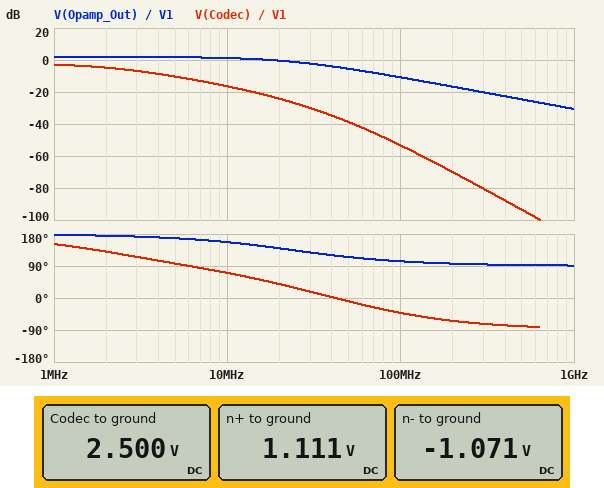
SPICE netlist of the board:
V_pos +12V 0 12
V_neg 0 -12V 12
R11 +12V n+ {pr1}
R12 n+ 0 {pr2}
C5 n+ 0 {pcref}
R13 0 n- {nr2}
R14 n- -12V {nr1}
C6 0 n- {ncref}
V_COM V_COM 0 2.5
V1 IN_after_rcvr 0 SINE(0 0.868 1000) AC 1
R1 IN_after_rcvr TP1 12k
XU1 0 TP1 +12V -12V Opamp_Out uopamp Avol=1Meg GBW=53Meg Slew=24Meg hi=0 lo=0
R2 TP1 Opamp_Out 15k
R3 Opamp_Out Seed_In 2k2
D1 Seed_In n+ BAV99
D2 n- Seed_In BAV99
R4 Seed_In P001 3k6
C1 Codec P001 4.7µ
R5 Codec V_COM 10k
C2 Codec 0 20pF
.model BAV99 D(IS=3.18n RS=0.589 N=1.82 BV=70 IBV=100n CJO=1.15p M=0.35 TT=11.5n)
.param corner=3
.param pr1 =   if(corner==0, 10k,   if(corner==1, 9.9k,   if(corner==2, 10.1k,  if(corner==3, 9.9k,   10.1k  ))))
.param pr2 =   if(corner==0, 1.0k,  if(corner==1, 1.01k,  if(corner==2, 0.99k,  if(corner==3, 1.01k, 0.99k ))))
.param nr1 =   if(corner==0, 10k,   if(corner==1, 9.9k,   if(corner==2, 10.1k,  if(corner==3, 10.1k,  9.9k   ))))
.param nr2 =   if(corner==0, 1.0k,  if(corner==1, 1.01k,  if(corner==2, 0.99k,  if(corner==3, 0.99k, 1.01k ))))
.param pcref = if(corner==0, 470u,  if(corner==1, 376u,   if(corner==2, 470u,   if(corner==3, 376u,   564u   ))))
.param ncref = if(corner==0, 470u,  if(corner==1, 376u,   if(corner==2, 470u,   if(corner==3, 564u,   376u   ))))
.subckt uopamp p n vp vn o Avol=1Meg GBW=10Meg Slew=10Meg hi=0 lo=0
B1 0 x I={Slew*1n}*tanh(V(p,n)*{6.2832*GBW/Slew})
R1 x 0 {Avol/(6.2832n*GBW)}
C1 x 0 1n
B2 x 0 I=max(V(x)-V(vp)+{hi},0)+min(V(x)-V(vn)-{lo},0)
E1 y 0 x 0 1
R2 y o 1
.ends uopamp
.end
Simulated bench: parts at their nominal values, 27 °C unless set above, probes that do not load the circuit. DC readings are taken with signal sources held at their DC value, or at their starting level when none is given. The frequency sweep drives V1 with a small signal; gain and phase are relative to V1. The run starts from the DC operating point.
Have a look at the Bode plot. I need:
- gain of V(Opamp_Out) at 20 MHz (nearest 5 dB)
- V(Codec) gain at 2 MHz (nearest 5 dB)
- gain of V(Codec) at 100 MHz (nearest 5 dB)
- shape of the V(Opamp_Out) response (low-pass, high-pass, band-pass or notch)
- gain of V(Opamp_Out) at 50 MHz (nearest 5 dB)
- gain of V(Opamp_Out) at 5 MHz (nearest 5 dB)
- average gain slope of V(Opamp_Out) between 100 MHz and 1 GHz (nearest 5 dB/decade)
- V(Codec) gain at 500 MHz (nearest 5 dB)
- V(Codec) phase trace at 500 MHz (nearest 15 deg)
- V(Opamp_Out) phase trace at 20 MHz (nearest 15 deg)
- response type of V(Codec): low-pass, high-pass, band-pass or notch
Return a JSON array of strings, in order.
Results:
["0 dB", "-5 dB", "-55 dB", "low-pass", "-5 dB", "0 dB", "-20 dB/decade", "-95 dB", "-75 deg", "135 deg", "low-pass"]
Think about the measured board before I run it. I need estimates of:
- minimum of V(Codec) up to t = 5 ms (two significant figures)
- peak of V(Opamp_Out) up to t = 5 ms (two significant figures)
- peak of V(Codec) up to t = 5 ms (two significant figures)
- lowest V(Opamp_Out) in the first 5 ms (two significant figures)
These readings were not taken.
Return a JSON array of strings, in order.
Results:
["1.8 V", "1.1 V", "3.2 V", "-1.1 V"]
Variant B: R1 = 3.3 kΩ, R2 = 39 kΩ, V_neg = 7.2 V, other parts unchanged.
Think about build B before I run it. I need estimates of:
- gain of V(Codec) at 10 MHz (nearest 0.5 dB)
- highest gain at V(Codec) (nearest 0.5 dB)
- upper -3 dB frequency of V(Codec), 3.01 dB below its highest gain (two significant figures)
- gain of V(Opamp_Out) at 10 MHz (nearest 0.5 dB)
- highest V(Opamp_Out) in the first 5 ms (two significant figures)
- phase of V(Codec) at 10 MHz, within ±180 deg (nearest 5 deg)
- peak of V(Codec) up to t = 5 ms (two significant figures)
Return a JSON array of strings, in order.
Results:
["-4.5 dB", "17.5 dB", "1.8 MHz", "13.0 dB", "10 V", "25 deg", "3.8 V"]
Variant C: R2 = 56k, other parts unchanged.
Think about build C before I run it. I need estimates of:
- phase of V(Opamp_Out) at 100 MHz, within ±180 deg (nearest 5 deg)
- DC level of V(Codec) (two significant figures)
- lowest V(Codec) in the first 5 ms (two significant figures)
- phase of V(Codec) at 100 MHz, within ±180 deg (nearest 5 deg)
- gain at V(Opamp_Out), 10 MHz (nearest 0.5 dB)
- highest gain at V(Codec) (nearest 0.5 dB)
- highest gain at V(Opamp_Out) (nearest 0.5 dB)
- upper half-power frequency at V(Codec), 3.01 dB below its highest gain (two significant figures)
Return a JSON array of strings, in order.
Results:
["95 deg", "2.5 V", "1.3 V", "-50 deg", "10.0 dB", "9.5 dB", "13.5 dB", "2.0 MHz"]
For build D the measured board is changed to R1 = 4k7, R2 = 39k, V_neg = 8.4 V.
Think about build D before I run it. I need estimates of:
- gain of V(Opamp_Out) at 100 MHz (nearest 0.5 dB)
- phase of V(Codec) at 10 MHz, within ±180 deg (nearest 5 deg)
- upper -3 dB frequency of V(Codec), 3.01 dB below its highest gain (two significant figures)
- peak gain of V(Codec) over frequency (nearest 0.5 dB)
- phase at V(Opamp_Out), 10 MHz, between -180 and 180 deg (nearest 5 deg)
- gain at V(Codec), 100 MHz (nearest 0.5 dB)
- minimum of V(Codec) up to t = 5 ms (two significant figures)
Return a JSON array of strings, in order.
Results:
["-6.5 dB", "35 deg", "1.9 MHz", "14.5 dB", "120 deg", "-49.0 dB", "1.5 V"]
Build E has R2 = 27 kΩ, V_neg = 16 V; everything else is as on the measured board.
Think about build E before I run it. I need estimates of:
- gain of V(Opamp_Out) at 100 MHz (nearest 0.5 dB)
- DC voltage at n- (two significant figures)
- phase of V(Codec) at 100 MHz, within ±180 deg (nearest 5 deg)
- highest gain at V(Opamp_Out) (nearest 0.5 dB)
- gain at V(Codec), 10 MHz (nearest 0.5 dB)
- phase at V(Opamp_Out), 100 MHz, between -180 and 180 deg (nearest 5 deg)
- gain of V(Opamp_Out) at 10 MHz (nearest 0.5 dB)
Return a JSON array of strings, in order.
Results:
["-9.0 dB", "-1.4 V", "-45 deg", "7.0 dB", "-12.0 dB", "100 deg", "5.5 dB"]
